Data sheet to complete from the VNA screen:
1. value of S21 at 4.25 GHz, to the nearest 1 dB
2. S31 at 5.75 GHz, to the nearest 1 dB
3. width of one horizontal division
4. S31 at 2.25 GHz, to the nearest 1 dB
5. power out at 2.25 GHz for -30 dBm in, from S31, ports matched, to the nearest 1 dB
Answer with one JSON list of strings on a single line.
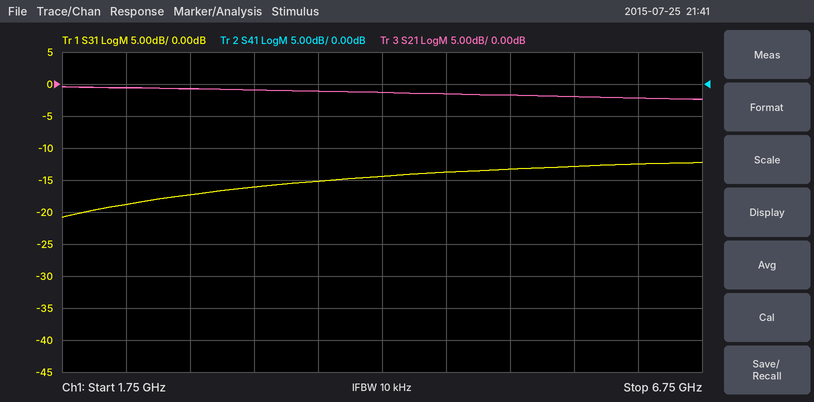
["-1 dB", "-13 dB", "500 MHz", "-19 dB", "-49 dBm"]
